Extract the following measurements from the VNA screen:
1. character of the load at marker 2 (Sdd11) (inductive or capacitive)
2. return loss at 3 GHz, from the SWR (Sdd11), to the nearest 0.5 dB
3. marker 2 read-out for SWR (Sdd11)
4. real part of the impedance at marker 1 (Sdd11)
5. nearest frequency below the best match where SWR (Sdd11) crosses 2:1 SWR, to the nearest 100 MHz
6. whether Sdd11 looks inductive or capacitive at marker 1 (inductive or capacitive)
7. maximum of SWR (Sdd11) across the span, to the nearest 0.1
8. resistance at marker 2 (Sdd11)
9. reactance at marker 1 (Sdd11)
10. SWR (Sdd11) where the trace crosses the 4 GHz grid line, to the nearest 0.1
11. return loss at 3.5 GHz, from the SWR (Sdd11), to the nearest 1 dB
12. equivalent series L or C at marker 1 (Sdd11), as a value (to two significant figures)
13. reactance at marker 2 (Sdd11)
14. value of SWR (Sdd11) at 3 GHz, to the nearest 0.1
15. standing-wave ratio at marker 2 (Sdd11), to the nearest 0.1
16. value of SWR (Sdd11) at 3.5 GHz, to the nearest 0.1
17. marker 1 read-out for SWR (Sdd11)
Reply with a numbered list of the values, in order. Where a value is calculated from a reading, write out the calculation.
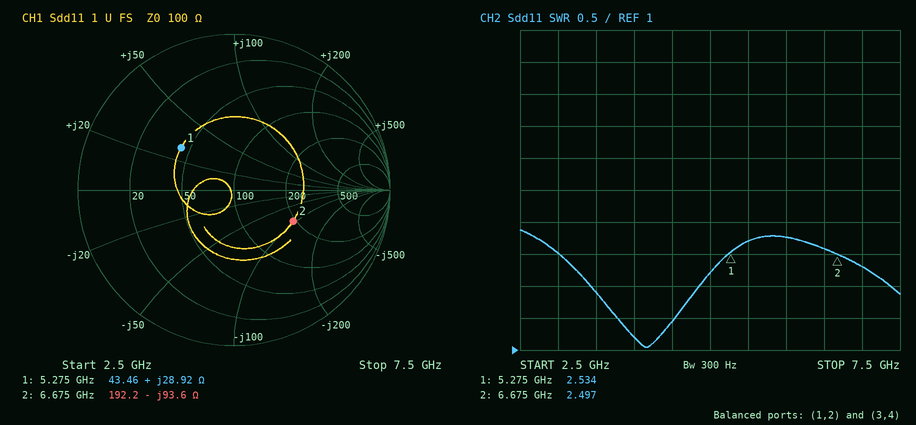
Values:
1. capacitive
2. −20 log10((2.5 − 1)/(2.5 + 1)) ≈ 7.36 dB, so 7.5 dB to the nearest 0.5 dB
3. 2.497
4. 43.46 Ω
5. 3.4 GHz
6. inductive
7. 2.9
8. 192.2 Ω
9. +28.92 Ω
10. 1.2
11. −20 log10((1.9 − 1)/(1.9 + 1)) ≈ 10 dB
12. L = 28.92 Ω/(2π × 5.275 GHz) ≈ 873 pH, so 870 pH to two significant figures
13. -93.6 Ω
14. 2.5
15. 2.5
16. 1.9
17. 2.534
